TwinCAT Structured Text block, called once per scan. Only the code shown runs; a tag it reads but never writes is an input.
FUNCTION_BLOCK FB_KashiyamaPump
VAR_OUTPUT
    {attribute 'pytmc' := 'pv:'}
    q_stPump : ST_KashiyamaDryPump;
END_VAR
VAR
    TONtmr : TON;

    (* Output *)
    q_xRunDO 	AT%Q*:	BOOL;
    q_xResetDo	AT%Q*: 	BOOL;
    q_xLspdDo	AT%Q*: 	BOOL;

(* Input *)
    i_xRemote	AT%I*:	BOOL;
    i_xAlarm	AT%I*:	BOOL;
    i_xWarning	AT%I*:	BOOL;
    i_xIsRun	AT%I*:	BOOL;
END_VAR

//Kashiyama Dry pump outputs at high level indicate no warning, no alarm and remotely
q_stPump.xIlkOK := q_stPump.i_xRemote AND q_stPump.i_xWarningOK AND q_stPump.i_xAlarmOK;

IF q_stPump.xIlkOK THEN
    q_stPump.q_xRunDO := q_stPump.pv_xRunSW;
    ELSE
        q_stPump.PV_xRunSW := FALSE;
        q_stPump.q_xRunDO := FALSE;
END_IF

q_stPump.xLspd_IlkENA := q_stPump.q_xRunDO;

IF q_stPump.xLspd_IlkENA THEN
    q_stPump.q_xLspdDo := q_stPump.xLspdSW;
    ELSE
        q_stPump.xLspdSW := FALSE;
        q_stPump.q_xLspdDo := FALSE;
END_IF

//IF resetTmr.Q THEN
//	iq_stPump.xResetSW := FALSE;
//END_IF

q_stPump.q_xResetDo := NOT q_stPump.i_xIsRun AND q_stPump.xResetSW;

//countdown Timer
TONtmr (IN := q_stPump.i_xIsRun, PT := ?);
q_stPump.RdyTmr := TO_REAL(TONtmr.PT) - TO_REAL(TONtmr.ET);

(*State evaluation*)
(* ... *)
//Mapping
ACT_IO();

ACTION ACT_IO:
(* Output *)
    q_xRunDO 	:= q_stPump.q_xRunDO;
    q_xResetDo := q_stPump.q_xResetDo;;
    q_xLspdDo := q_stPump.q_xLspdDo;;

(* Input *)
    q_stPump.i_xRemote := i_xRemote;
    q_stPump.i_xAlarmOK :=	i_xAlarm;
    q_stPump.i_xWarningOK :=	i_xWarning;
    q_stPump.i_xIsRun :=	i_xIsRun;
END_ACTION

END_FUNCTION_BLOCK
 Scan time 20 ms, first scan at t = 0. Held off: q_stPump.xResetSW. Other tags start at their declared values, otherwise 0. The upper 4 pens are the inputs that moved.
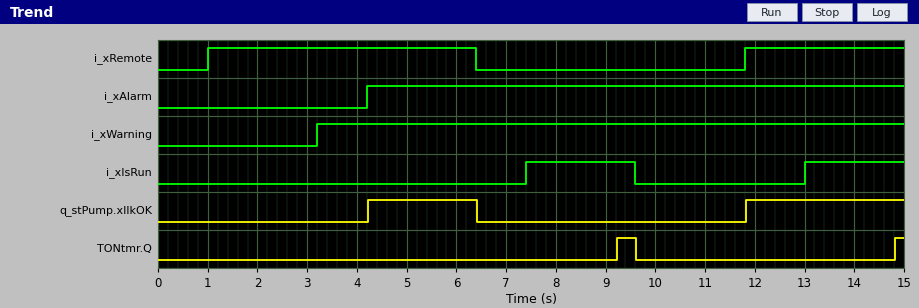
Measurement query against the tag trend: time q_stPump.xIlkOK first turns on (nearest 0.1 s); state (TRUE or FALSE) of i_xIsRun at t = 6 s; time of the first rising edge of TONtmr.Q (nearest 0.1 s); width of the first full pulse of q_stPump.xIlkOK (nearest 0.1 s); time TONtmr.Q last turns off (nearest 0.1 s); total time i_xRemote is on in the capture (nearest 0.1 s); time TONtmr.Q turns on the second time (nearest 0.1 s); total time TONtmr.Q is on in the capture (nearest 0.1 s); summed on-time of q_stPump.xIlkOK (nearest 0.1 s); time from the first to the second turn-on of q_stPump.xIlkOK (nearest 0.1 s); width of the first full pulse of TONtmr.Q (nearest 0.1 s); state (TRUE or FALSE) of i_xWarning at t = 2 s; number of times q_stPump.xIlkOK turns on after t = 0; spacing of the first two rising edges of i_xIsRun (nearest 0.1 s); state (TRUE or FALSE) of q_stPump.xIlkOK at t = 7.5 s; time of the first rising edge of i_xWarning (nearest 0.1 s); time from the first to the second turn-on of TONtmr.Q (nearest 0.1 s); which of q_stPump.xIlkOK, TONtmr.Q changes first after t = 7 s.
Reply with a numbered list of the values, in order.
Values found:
1. 4.2 s
2. FALSE
3. 9.2 s
4. 2.2 s
5. 9.6 s
6. 8.6 s
7. 14.8 s
8. 0.6 s
9. 5.4 s
10. 7.6 s
11. 0.4 s
12. FALSE
13. 2
14. 5.6 s
15. FALSE
16. 3.2 s
17. 5.6 s
18. TONtmr.Q
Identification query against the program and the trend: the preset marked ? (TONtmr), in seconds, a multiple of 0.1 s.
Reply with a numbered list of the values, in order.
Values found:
1. 1.8 s
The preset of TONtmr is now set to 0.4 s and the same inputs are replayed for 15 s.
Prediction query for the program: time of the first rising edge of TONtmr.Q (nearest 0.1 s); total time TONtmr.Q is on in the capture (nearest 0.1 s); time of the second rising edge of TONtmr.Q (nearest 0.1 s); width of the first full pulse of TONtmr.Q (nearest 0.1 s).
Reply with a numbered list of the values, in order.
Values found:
1. 7.8 s
2. 3.4 s
3. 13.4 s
4. 1.8 s
